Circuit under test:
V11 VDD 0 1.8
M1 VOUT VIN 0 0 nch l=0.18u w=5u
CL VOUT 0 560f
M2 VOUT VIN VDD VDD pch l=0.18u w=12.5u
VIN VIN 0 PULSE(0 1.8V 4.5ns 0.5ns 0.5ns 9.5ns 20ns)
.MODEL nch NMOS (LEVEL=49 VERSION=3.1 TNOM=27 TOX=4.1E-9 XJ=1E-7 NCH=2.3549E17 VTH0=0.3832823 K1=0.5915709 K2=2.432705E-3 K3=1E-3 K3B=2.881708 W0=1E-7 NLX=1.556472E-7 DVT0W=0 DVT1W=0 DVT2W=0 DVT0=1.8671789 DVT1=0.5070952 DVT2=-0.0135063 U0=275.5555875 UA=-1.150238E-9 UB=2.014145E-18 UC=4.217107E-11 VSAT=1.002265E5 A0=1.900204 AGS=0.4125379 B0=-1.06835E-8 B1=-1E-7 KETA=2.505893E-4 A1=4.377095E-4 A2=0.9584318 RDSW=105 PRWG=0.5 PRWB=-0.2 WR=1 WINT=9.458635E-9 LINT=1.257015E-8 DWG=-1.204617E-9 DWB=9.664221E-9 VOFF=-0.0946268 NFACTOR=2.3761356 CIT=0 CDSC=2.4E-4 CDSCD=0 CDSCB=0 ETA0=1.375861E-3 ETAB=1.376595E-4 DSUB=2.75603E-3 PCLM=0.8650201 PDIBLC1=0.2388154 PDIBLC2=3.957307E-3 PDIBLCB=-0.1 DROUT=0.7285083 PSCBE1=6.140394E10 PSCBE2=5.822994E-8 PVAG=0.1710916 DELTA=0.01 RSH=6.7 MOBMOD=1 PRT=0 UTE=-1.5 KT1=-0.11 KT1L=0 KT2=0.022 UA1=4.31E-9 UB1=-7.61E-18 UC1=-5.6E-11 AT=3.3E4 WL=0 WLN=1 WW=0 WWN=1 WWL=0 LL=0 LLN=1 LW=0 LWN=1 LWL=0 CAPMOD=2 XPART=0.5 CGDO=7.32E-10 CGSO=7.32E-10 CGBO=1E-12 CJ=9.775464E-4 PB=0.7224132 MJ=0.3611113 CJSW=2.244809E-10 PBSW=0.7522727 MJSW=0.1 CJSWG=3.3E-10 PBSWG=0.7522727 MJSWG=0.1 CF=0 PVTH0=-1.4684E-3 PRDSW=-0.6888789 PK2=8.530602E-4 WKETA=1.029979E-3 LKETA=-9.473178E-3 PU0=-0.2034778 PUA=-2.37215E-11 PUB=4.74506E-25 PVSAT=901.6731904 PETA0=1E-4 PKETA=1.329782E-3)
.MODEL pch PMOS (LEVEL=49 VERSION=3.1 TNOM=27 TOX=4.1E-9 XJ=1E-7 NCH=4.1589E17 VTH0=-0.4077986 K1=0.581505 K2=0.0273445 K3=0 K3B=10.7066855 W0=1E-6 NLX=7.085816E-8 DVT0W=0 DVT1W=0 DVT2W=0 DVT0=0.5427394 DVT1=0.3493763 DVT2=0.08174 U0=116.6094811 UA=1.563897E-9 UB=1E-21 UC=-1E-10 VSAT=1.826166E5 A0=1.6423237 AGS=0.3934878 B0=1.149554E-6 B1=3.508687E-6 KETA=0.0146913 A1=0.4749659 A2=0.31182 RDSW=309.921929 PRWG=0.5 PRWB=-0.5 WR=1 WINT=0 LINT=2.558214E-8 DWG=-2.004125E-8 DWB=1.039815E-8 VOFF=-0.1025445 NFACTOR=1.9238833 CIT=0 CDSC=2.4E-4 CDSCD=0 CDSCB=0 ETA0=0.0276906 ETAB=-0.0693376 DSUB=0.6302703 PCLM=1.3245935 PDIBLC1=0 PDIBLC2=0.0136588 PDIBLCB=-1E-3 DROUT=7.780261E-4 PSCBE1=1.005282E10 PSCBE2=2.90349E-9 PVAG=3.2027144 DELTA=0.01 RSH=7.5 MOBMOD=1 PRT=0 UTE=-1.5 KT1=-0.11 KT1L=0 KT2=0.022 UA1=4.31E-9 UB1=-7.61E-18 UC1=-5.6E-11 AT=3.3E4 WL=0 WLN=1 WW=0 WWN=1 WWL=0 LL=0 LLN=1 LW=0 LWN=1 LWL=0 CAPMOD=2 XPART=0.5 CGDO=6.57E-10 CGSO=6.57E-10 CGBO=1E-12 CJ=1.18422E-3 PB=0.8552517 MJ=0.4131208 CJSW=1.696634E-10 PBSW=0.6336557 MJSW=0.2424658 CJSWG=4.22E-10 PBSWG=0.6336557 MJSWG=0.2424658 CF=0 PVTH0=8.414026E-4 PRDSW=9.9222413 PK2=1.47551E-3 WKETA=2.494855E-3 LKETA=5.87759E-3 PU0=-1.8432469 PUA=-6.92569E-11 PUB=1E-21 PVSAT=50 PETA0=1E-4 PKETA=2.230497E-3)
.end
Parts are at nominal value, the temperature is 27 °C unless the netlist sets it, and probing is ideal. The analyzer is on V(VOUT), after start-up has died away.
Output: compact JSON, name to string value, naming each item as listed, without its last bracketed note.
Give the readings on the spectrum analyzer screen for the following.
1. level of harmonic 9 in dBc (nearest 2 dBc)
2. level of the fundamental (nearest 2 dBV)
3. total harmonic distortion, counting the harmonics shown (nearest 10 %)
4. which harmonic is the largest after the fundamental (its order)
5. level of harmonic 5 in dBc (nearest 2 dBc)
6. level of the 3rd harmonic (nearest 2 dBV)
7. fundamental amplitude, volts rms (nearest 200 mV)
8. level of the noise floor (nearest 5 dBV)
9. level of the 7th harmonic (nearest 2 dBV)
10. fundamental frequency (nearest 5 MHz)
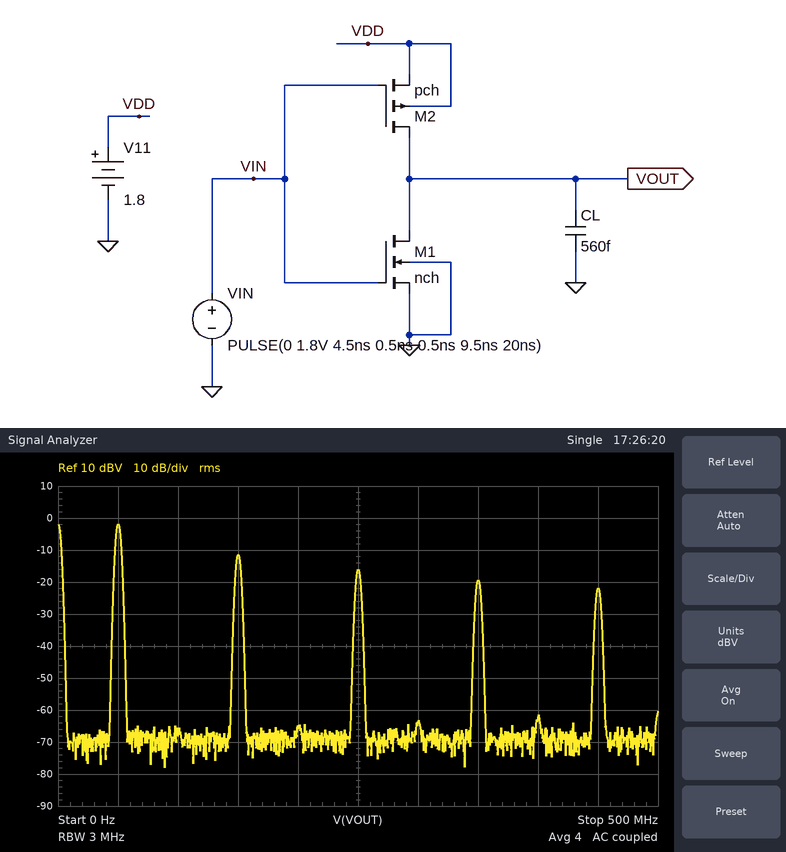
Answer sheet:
{"level of harmonic 9 in dBc": "-20 dBc", "level of the fundamental": "-2 dBV", "total harmonic distortion, counting the harmonics shown": "40 %", "which harmonic is the largest after the fundamental": "3", "level of harmonic 5 in dBc": "-14 dBc", "level of the 3rd harmonic": "-12 dBV", "fundamental amplitude, volts rms": "800 mV", "level of the noise floor": "-70 dBV", "level of the 7th harmonic": "-20 dBV", "fundamental frequency": "50 MHz"}
